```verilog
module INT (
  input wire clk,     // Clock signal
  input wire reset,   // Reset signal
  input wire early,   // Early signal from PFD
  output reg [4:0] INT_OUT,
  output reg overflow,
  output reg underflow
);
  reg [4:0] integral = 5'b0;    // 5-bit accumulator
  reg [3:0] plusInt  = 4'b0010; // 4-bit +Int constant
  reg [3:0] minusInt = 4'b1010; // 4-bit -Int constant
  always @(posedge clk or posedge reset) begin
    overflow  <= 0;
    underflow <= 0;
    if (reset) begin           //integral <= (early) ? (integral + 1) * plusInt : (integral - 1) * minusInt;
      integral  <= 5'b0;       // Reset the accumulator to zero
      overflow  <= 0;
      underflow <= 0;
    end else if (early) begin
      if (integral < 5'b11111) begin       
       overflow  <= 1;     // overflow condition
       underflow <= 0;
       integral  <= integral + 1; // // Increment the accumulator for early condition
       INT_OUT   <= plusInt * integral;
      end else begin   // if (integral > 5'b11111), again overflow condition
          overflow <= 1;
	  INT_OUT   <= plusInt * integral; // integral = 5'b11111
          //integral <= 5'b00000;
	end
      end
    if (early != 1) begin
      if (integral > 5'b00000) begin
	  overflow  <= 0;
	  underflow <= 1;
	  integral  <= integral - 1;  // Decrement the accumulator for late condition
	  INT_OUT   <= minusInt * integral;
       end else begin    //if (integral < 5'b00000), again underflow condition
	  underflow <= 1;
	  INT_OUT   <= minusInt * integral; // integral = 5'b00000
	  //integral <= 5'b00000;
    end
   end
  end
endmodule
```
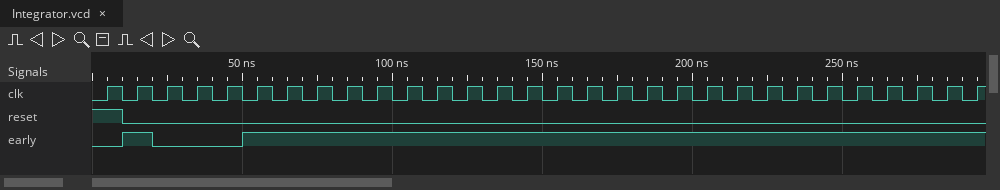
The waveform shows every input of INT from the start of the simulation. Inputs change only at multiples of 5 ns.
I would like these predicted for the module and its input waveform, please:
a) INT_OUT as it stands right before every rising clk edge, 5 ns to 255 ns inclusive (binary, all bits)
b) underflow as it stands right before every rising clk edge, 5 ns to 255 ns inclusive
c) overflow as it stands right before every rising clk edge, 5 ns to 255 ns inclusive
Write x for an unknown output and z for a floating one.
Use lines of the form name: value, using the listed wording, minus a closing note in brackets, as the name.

INT_OUT as it stands right before every rising clk edge, 5 ns to 255 ns inclusive: 00000, 00000, 00000, 01010, 00000, 00000, 00000, 00010, 00100, 00110, 01000, 01010, 01100, 01110, 10000, 10010, 10100, 10110, 11000, 11010, 11100, 11110, 00000, 00010, 00100, 00110
underflow as it stands right before every rising clk edge, 5 ns to 255 ns inclusive: 1 1 0 1 1 1 0 0 0 0 0 0 0 0 0 0 0 0 0 0 0 0 0 0 0 0
overflow as it stands right before every rising clk edge, 5 ns to 255 ns inclusive: 0 0 1 0 0 0 1 1 1 1 1 1 1 1 1 1 1 1 1 1 1 1 1 1 1 1
